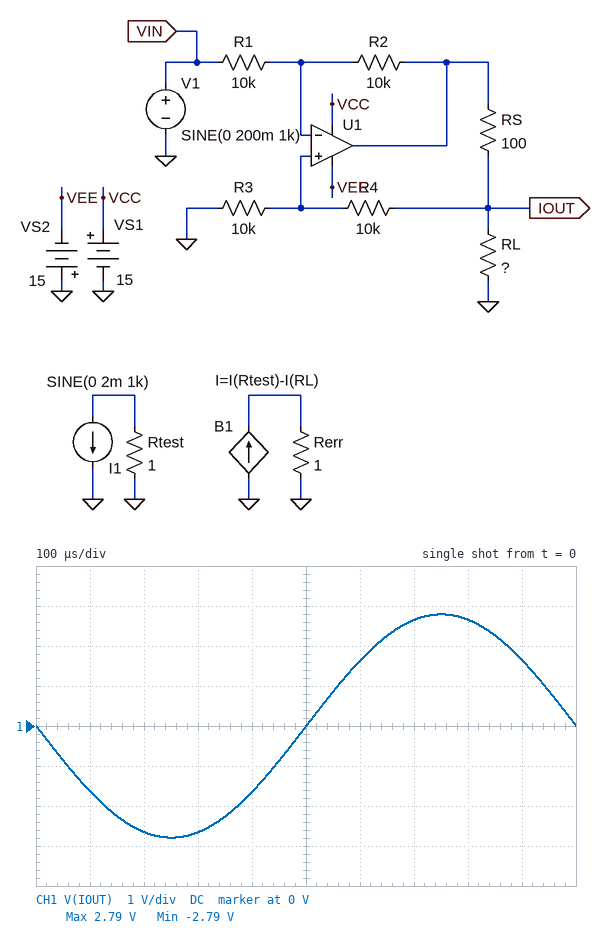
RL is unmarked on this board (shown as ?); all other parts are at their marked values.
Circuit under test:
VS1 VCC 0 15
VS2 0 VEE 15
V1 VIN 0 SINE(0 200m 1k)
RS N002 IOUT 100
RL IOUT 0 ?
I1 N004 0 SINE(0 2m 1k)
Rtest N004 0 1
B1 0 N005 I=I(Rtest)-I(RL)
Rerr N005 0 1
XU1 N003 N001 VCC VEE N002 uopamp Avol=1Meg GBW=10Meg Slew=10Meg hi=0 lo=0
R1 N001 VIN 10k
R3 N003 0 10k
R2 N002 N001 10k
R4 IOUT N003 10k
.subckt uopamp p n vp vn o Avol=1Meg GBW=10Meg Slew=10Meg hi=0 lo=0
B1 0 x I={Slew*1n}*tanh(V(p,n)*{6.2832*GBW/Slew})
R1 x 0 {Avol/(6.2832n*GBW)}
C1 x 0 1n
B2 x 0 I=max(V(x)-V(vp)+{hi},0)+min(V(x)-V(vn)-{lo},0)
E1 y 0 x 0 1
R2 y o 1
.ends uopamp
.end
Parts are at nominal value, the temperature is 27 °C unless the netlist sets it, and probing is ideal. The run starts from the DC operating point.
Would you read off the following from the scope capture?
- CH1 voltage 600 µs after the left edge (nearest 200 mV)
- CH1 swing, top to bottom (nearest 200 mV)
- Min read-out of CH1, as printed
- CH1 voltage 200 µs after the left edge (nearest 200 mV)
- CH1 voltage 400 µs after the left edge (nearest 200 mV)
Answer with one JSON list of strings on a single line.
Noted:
["1.6 V", "5.6 V", "-2.79 V", "-2.6 V", "-1.6 V"]
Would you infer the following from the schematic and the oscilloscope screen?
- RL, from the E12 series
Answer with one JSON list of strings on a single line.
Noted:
["1.5 kΩ"]
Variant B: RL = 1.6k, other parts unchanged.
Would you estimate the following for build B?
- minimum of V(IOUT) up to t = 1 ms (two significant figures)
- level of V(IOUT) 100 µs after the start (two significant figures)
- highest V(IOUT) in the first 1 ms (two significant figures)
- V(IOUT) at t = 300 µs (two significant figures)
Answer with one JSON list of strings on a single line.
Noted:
["-3.0 V", "-1.7 V", "3.0 V", "-2.8 V"]
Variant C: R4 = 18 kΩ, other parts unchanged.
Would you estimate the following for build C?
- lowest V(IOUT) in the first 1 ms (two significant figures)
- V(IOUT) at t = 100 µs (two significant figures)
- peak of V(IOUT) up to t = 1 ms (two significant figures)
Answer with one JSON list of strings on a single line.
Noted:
["-560 mV", "-330 mV", "560 mV"]
